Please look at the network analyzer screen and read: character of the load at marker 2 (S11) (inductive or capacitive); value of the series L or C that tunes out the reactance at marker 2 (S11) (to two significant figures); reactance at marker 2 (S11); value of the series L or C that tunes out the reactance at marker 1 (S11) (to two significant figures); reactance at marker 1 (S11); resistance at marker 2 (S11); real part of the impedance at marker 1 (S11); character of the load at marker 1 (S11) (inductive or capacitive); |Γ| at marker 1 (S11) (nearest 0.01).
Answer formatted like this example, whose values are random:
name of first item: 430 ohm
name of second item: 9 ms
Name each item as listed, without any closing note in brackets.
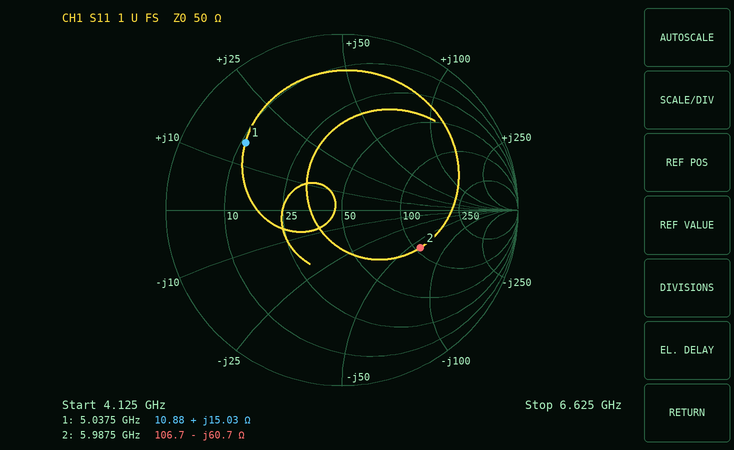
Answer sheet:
character of the load at marker 2 (S11): capacitive
value of the series L or C that tunes out the reactance at marker 2 (S11): 1.6 nH
reactance at marker 2: -60.7 Ω
value of the series L or C that tunes out the reactance at marker 1 (S11): 2.1 pF
reactance at marker 1: +15.03 Ω
resistance at marker 2: 106.7 Ω
real part of the impedance at marker 1: 10.88 Ω
character of the load at marker 1 (S11): inductive
|Γ| at marker 1 (S11): 0.67
